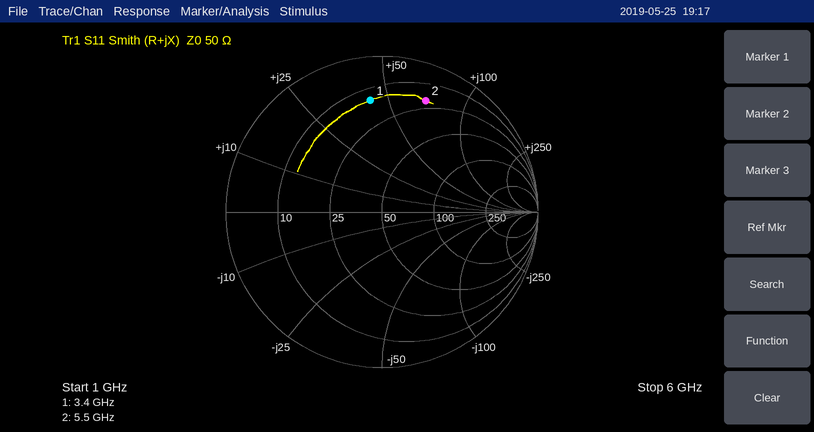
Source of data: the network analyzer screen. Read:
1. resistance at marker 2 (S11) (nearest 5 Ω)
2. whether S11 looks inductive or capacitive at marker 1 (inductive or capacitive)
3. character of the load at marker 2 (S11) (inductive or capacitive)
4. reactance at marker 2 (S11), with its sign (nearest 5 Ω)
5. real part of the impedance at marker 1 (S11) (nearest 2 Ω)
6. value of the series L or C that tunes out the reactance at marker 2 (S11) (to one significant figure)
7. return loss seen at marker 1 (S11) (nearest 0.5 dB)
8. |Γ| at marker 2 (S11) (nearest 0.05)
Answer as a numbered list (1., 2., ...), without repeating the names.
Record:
1. 20 Ω
2. inductive
3. inductive
4. +70 Ω
5. 14 Ω
6. 400 fF
7. 3.0 dB
8. 0.75
